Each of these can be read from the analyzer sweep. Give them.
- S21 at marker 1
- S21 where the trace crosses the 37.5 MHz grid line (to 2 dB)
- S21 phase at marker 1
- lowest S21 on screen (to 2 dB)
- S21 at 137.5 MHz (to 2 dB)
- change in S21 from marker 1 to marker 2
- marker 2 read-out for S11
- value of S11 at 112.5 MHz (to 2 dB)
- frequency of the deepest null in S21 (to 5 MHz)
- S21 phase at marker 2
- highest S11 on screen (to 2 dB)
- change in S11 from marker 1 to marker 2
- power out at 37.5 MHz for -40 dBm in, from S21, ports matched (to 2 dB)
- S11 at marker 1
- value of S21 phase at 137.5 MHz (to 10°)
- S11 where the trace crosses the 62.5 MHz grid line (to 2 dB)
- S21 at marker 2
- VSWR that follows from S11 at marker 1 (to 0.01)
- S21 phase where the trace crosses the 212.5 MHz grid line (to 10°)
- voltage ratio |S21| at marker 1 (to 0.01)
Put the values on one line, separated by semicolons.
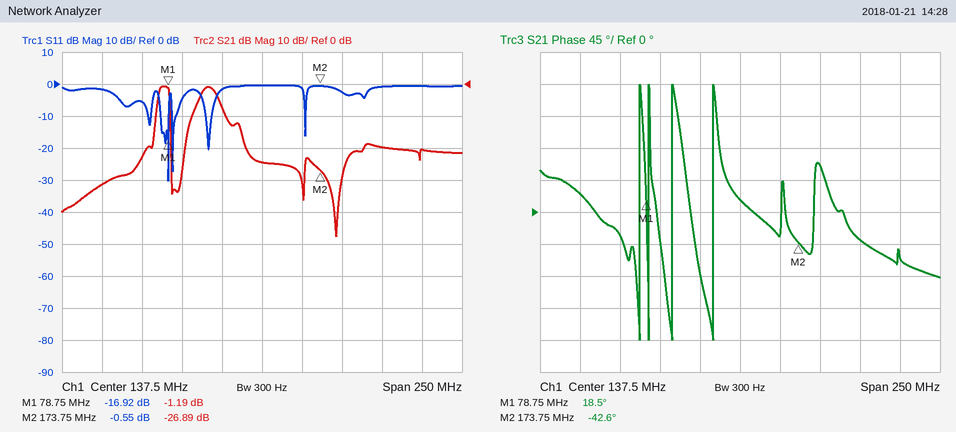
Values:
-1.19 dB; -32 dB; 18.5°; -48 dB; -24 dB; -25.70 dB; -0.55 dB; -2 dB; 185 MHz; -42.6°; 0 dB; 16.37 dB; -72 dBm; -16.92 dB; 20°; -6 dB; -26.89 dB; 1.33; -40°; 0.87
